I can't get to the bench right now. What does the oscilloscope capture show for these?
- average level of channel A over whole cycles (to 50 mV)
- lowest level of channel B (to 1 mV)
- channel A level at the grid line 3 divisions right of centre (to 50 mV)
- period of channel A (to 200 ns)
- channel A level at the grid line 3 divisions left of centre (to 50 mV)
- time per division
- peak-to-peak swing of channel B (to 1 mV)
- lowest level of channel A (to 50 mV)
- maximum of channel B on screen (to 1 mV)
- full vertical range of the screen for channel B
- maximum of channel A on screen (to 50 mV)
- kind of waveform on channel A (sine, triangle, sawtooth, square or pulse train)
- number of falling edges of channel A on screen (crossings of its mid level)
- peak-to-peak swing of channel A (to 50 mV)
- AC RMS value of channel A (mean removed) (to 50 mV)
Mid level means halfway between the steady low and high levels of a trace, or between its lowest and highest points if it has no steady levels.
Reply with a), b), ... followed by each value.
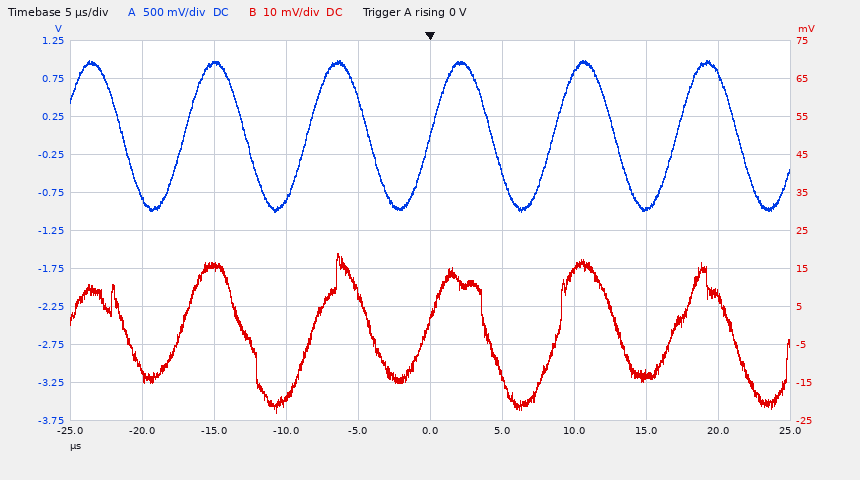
a) 0 mV
b) -23 mV
c) -950 mV
d) 8.6 µs
e) 950 mV
f) 5 µs
g) 42 mV
h) -1.00 V
i) 19 mV
j) 100 mV
k) 1.00 V
l) sine
m) 6
n) 2.00 V
o) 700 mV
